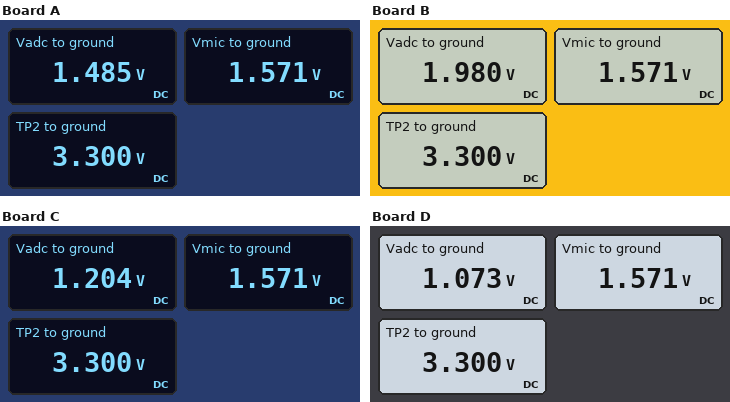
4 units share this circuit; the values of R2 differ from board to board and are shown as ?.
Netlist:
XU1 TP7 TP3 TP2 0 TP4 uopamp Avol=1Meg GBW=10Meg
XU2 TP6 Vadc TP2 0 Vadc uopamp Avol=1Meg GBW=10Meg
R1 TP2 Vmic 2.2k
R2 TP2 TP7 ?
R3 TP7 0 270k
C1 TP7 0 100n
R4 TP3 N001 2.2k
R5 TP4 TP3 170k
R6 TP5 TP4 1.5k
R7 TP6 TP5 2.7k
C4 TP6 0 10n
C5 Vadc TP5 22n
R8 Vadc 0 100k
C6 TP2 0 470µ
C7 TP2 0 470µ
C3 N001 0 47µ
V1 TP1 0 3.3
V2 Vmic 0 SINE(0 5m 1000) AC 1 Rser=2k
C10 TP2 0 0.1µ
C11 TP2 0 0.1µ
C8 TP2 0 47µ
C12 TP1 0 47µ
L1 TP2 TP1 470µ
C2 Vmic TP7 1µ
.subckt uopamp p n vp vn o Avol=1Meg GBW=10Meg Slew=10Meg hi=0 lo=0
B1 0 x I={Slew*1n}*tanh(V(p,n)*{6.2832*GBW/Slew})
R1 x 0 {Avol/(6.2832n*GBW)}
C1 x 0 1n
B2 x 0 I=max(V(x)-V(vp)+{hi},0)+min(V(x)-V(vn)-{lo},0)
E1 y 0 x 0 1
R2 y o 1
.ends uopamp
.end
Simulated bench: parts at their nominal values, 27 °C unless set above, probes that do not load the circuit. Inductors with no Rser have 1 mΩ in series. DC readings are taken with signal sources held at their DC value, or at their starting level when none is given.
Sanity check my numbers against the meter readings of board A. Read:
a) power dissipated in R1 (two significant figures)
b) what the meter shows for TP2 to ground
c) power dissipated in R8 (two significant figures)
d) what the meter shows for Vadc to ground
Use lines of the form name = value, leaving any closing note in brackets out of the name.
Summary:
power dissipated in R1 = 1.4 mW
what the meter shows for TP2 to ground = 3.300 V
power dissipated in R8 = 22 µW
what the meter shows for Vadc to ground = 1.485 V
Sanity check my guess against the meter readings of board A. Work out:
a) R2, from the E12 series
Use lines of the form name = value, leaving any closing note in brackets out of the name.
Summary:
R2, from the E12 series = 330 kΩ
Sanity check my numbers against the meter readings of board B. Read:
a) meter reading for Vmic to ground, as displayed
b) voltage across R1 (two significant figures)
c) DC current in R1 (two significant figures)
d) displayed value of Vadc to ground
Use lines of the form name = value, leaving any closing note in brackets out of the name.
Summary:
meter reading for Vmic to ground, as displayed = 1.571 V
voltage across R1 = 1.7 V
DC current in R1 = 790 µA
displayed value of Vadc to ground = 1.980 V
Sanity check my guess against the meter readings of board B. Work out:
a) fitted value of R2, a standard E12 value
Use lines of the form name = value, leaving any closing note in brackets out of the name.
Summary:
fitted value of R2, a standard E12 value = 180 kΩ
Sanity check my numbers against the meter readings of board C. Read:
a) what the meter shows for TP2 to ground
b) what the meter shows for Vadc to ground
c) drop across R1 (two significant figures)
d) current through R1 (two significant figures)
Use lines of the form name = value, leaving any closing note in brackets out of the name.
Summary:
what the meter shows for TP2 to ground = 3.300 V
what the meter shows for Vadc to ground = 1.204 V
drop across R1 = 1.7 V
current through R1 = 790 µA
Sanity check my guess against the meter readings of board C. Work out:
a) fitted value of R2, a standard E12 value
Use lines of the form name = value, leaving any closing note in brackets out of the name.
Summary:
fitted value of R2, a standard E12 value = 470 kΩ
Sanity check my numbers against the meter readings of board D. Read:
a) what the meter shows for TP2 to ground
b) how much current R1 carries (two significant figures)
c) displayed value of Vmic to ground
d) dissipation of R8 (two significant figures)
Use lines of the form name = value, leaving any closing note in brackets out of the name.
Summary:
what the meter shows for TP2 to ground = 3.300 V
how much current R1 carries = 790 µA
displayed value of Vmic to ground = 1.571 V
dissipation of R8 = 12 µW
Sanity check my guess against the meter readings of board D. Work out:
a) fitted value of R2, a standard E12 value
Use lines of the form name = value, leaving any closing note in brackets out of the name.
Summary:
fitted value of R2, a standard E12 value = 560 kΩ
